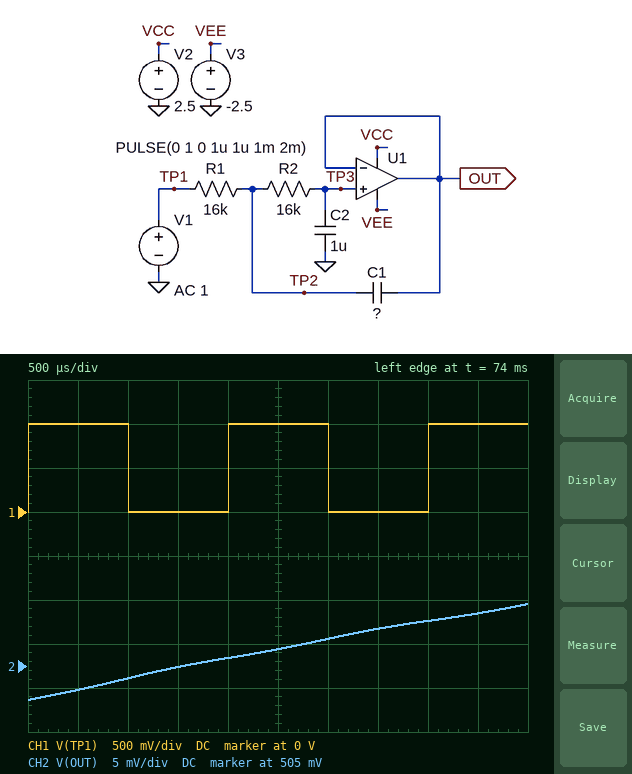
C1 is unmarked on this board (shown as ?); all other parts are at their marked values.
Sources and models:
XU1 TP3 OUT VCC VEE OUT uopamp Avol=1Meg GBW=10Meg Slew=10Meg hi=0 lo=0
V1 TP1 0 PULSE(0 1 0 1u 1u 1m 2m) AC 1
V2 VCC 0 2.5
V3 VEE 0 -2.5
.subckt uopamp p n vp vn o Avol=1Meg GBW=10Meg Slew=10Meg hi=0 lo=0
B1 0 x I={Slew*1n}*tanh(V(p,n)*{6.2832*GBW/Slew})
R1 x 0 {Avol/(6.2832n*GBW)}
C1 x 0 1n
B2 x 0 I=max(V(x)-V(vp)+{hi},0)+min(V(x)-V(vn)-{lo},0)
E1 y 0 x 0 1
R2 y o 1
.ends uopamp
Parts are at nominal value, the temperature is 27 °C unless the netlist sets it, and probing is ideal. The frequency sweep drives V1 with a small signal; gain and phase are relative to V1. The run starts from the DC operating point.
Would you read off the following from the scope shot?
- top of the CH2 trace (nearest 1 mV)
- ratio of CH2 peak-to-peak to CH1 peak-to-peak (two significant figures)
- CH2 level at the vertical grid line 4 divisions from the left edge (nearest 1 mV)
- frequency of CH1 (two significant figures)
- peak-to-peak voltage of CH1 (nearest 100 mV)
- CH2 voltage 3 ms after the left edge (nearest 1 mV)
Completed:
512 mV
0.011
506 mV
500 Hz
1.0 V
508 mV
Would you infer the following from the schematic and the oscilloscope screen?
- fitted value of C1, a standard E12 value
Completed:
2.2 µF
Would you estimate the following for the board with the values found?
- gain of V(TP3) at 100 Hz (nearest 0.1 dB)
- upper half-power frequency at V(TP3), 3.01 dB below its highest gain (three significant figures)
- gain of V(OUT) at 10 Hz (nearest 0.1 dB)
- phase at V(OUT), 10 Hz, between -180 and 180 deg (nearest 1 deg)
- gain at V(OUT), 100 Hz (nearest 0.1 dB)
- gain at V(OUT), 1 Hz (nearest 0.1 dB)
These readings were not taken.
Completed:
-46.9 dB
6.99 Hz
-7.4 dB
-121 deg
-46.9 dB
0 dB
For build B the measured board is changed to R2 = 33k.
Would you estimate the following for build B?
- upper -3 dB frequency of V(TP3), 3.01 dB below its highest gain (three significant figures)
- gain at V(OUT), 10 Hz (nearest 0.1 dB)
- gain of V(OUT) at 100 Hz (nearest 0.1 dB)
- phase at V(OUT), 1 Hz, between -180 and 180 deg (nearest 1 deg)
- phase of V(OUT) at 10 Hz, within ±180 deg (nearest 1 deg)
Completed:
4.59 Hz
-13.5 dB
-53.2 dB
-18 deg
-139 deg
